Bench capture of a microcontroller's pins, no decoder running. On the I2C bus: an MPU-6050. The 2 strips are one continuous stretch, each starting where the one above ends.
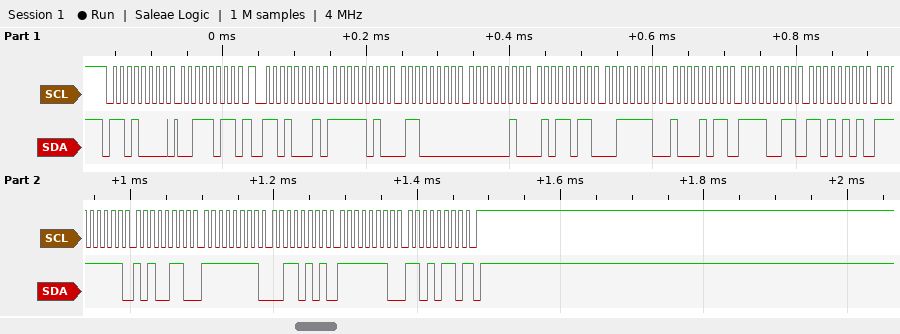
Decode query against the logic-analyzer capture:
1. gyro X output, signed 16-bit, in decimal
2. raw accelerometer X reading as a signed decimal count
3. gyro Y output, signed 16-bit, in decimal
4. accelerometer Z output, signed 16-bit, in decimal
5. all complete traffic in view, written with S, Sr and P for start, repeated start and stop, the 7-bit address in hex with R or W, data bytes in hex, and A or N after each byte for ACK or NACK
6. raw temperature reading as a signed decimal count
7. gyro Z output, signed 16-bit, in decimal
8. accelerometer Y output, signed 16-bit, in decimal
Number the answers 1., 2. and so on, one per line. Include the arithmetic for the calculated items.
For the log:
1. 0xFFA6 = -90
2. 0xFA60 = -1440
3. 0xFF35 = -203
4. 0x3E8B = 16011
5. S 68W A 3B A Sr 68R A FA A 60 A 02 A 5B A 3E A 8B A F3 A D5 A FF A A6 A FF A 35 A FE A D6 N P
6. 0xF3D5 = -3115
7. 0xFED6 = -298
8. 0x025B = 603
